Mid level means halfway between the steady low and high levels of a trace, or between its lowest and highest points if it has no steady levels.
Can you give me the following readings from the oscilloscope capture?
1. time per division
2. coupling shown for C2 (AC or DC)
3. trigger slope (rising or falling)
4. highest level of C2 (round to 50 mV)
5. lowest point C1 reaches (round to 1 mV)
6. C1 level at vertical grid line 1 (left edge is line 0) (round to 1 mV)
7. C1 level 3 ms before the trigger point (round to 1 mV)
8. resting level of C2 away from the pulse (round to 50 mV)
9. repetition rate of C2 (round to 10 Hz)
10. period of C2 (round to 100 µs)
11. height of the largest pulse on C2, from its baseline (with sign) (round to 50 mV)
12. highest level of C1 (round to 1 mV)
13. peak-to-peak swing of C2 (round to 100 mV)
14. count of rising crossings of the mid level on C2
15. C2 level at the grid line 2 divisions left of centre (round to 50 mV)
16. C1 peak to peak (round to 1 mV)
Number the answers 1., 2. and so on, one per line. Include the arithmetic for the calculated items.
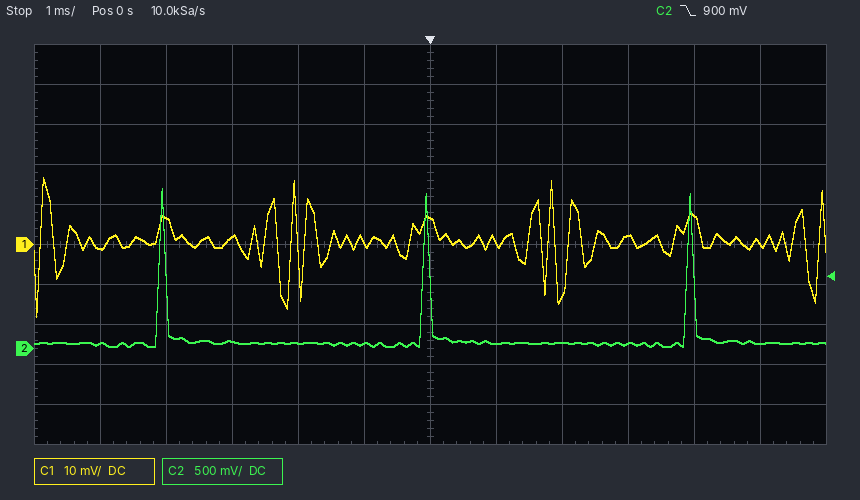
1. 1 ms
2. DC
3. falling
4. 2.00 V
5. -18 mV
6. -1 mV
7. 2 mV
8. 50 mV
9. 1 / 4.0 ms ≈ 250 Hz
10. 4.0 ms
11. 2.00 V − (50 mV) = +1.95 V
12. 17 mV
13. 2.00 V
14. 3
15. 50 mV
16. 17 mV − (-18 mV) = 35 mV
